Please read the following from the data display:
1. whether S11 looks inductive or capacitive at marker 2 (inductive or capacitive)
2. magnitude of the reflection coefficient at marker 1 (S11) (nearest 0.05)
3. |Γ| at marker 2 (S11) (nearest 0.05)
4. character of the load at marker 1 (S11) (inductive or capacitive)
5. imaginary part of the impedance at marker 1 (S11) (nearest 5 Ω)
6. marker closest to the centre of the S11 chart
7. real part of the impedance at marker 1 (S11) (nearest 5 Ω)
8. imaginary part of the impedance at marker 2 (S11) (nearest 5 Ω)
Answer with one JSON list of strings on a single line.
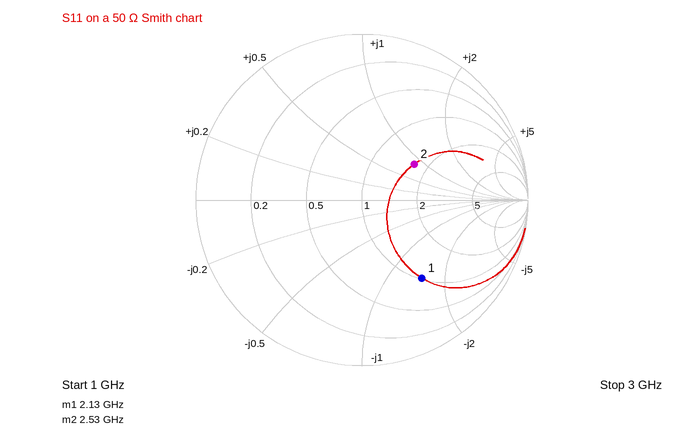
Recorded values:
["inductive", "0.60", "0.40", "capacitive", "-75 Ω", "marker 2", "50 Ω", "+40 Ω"]
